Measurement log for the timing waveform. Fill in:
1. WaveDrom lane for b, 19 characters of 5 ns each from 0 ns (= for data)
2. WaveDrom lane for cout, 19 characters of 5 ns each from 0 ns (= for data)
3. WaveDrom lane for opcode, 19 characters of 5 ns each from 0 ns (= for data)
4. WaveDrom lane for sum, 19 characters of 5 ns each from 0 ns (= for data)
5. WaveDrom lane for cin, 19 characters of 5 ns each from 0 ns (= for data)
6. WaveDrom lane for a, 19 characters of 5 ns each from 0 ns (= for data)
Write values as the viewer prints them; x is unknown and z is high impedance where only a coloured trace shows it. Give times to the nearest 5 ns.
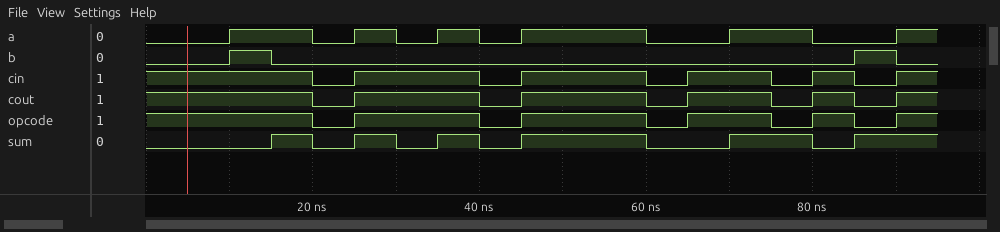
{name: 'b', wave: '0.10.............10'}
{name: 'cout', wave: '1...01..01..01.0101'}
{name: 'opcode', wave: '1...01..01..01.0101'}
{name: 'sum', wave: '0..1010101..0.1.01.'}
{name: 'cin', wave: '1...01..01..01.0101'}
{name: 'a', wave: '0.1.010101..0.1.0.1'}
